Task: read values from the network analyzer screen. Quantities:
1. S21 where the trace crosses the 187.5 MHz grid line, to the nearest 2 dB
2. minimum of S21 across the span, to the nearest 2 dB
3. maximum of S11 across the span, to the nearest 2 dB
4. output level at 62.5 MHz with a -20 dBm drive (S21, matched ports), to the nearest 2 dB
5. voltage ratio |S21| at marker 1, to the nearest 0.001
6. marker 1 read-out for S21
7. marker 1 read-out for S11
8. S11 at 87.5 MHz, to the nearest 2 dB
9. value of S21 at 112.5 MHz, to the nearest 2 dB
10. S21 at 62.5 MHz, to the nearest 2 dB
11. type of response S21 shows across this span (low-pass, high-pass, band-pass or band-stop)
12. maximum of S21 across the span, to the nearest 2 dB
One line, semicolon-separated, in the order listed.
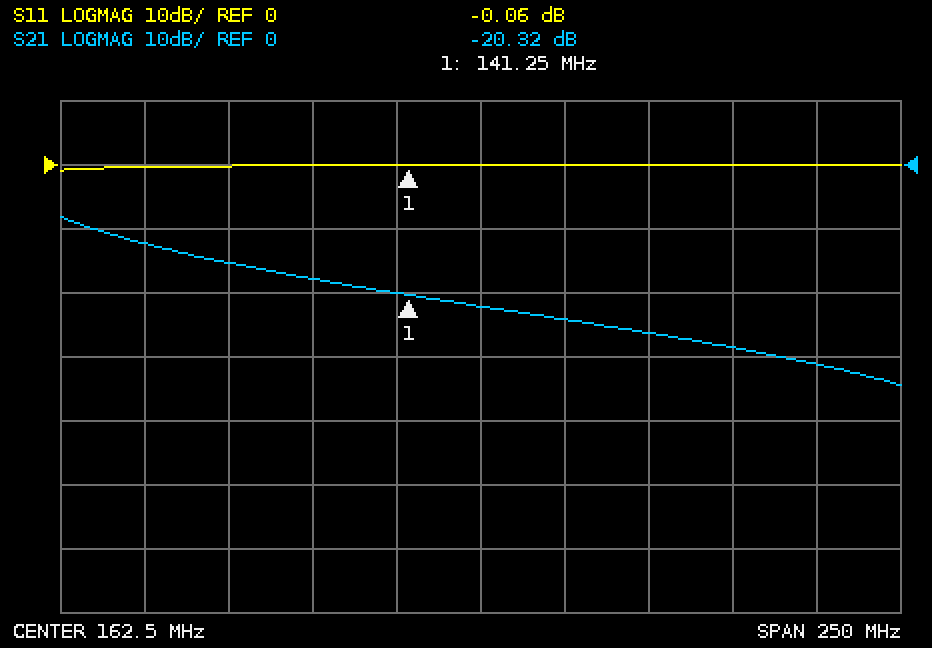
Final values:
-24 dB; -34 dB; 0 dB; -32 dBm; 0.096; -20.32 dB; -0.06 dB; 0 dB; -18 dB; -12 dB; low-pass; -8 dB
